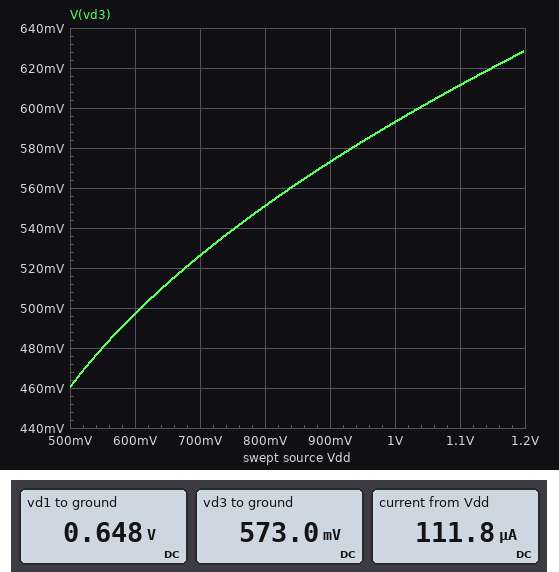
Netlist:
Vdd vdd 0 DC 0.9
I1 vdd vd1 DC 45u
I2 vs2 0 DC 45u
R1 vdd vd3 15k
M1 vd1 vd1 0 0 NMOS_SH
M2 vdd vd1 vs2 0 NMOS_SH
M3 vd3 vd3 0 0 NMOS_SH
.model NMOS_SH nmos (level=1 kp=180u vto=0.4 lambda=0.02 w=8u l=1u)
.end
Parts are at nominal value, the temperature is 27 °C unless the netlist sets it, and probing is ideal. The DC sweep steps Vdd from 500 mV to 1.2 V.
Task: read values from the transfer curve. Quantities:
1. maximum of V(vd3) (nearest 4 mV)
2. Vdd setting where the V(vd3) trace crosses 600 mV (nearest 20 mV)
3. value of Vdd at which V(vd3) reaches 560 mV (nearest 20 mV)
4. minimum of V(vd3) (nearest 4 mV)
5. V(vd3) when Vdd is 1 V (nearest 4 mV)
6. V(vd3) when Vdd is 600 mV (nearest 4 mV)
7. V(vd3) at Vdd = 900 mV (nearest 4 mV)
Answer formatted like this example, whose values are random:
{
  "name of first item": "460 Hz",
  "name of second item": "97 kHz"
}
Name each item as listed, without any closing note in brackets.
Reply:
{
  "maximum of V(vd3)": "628 mV",
  "Vdd setting where the V(vd3) trace crosses 600 mV": "1.04 V",
  "value of Vdd at which V(vd3) reaches 560 mV": "840 mV",
  "minimum of V(vd3)": "460 mV",
  "V(vd3) when Vdd is 1 V": "592 mV",
  "V(vd3) when Vdd is 600 mV": "496 mV",
  "V(vd3) at Vdd = 900 mV": "572 mV"
}
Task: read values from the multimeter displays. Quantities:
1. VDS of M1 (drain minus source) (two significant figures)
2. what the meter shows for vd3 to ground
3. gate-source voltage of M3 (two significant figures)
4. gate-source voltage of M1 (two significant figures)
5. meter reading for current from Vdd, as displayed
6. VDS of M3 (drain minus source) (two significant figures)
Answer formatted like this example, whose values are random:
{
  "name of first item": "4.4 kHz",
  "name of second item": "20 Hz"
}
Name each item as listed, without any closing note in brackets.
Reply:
{
  "VDS of M1 (drain minus source)": "650 mV",
  "what the meter shows for vd3 to ground": "573.0 mV",
  "gate-source voltage of M3": "570 mV",
  "gate-source voltage of M1": "650 mV",
  "meter reading for current from Vdd, as displayed": "111.8 µA",
  "VDS of M3 (drain minus source)": "570 mV"
}
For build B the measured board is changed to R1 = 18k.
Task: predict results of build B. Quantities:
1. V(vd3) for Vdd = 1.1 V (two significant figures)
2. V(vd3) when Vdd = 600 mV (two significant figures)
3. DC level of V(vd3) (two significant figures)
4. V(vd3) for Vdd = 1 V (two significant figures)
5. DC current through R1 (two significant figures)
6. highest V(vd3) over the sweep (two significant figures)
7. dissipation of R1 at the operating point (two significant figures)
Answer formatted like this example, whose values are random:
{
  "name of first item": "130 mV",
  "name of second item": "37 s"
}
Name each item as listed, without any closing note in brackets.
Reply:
{
  "V(vd3) for Vdd = 1.1 V": "600 mV",
  "V(vd3) when Vdd = 600 mV": "490 mV",
  "DC level of V(vd3)": "560 mV",
  "V(vd3) for Vdd = 1 V": "580 mV",
  "DC current through R1": "19 µA",
  "highest V(vd3) over the sweep": "610 mV",
  "dissipation of R1 at the operating point": "6.4 µW"
}
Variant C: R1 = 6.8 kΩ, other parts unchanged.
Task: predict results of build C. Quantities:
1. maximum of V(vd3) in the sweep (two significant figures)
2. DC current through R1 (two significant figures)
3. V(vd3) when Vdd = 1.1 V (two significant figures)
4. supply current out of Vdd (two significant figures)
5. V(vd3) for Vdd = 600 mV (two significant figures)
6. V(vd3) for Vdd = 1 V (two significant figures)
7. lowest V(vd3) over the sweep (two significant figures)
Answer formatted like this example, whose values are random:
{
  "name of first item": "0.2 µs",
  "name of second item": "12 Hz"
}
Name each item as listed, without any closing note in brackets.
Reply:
{
  "maximum of V(vd3) in the sweep": "710 mV",
  "DC current through R1": "39 µA",
  "V(vd3) when Vdd = 1.1 V": "690 mV",
  "supply current out of Vdd": "130 µA",
  "V(vd3) for Vdd = 600 mV": "520 mV",
  "V(vd3) for Vdd = 1 V": "660 mV",
  "lowest V(vd3) over the sweep": "470 mV"
}
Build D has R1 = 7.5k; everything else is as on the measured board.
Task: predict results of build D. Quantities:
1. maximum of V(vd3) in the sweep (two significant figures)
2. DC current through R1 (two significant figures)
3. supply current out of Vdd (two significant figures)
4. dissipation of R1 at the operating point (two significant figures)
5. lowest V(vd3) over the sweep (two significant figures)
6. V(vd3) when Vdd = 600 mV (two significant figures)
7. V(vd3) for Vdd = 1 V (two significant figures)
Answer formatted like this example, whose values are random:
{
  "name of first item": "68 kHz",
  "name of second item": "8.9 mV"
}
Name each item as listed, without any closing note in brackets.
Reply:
{
  "maximum of V(vd3) in the sweep": "700 mV",
  "DC current through R1": "37 µA",
  "supply current out of Vdd": "130 µA",
  "dissipation of R1 at the operating point": "10 µW",
  "lowest V(vd3) over the sweep": "470 mV",
  "V(vd3) when Vdd = 600 mV": "520 mV",
  "V(vd3) for Vdd = 1 V": "650 mV"
}
